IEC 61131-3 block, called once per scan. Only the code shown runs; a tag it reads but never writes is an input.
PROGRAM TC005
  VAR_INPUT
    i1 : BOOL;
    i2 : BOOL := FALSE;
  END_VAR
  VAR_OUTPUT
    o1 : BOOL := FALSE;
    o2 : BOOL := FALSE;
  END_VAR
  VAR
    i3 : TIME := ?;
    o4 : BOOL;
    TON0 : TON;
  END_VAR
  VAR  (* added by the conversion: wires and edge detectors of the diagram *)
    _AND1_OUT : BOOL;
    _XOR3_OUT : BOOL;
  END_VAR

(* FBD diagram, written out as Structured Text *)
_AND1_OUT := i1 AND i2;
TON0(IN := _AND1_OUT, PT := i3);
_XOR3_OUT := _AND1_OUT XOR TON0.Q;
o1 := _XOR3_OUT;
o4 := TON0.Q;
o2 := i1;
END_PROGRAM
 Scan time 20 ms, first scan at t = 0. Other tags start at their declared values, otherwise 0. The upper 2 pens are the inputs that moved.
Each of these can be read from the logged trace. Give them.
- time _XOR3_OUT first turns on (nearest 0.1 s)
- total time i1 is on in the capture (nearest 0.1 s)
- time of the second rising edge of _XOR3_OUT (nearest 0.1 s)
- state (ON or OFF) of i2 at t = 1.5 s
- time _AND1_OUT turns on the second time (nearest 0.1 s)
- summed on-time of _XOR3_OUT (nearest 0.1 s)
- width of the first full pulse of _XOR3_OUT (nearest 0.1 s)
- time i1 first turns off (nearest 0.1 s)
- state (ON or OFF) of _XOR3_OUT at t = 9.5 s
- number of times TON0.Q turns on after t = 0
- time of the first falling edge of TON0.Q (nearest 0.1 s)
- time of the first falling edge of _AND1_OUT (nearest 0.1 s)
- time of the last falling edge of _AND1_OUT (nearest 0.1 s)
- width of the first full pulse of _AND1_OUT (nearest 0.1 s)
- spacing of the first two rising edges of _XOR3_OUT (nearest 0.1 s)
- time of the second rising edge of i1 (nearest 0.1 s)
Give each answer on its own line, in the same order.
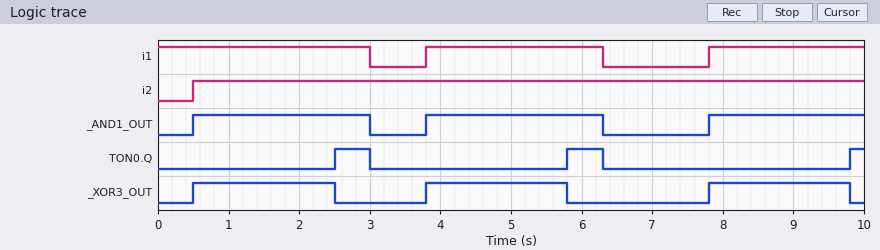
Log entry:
0.5 s
7.7 s
3.8 s
ON
3.8 s
6.0 s
2.0 s
3.0 s
ON
3
3.0 s
3.0 s
6.3 s
2.5 s
3.3 s
7.8 s
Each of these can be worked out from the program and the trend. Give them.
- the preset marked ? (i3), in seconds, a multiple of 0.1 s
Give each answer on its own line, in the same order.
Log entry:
2.0 s
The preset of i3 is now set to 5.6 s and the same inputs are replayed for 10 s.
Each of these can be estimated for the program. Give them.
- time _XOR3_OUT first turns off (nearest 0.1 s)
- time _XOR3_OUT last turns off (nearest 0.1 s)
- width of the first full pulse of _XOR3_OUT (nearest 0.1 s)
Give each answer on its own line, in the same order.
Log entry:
3.0 s
6.3 s
2.5 s
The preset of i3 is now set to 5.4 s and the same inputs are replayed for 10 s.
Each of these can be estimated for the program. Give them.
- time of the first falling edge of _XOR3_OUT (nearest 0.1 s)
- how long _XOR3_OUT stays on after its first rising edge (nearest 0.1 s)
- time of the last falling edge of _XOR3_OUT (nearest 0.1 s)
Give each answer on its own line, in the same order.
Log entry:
3.0 s
2.5 s
6.3 s
